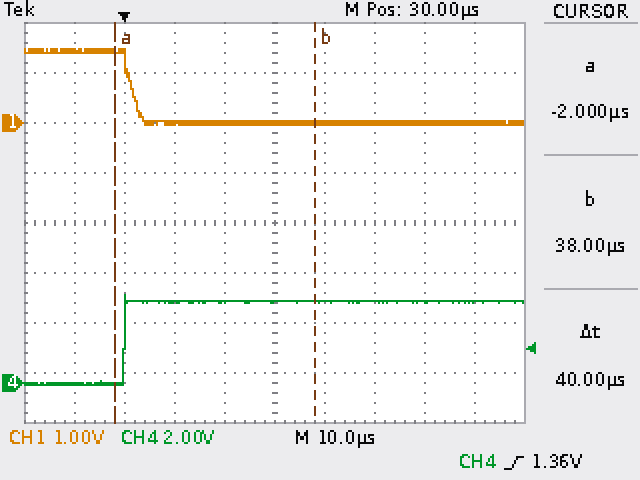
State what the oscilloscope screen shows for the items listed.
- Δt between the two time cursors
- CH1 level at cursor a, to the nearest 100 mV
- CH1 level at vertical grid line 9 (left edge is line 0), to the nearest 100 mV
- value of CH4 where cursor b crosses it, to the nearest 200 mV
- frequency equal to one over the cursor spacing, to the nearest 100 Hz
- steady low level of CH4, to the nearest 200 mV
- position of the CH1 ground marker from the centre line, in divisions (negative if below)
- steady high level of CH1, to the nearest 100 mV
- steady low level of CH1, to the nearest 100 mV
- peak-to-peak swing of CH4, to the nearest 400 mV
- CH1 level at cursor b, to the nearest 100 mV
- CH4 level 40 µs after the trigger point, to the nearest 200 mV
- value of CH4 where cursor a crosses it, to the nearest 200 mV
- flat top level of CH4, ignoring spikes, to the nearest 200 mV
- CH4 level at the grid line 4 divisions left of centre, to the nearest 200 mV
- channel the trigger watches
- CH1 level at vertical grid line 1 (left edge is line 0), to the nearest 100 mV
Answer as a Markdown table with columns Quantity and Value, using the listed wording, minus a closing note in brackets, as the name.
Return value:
| Quantity | Value |
|---|---|
| Δt between the two time cursors | 40 µs |
| CH1 level at cursor a, to the nearest 100 mV | 1.4 V |
| CH1 level at vertical grid line 9 (left edge is line 0), to the nearest 100 mV | 0.0 V |
| value of CH4 where cursor b crosses it, to the nearest 200 mV | 3.2 V |
| frequency equal to one over the cursor spacing, to the nearest 100 Hz | 25.0 kHz |
| steady low level of CH4, to the nearest 200 mV | 0.0 V |
| position of the CH1 ground marker from the centre line, in divisions | +2.0 div |
| steady high level of CH1, to the nearest 100 mV | 1.4 V |
| steady low level of CH1, to the nearest 100 mV | 0.0 V |
| peak-to-peak swing of CH4, to the nearest 400 mV | 3.6 V |
| CH1 level at cursor b, to the nearest 100 mV | 0.0 V |
| CH4 level 40 µs after the trigger point, to the nearest 200 mV | 3.2 V |
| value of CH4 where cursor a crosses it, to the nearest 200 mV | 0.0 V |
| flat top level of CH4, ignoring spikes, to the nearest 200 mV | 3.2 V |
| CH4 level at the grid line 4 divisions left of centre, to the nearest 200 mV | 0.0 V |
| channel the trigger watches | CH4 |
| CH1 level at vertical grid line 1 (left edge is line 0), to the nearest 100 mV | 1.4 V |
